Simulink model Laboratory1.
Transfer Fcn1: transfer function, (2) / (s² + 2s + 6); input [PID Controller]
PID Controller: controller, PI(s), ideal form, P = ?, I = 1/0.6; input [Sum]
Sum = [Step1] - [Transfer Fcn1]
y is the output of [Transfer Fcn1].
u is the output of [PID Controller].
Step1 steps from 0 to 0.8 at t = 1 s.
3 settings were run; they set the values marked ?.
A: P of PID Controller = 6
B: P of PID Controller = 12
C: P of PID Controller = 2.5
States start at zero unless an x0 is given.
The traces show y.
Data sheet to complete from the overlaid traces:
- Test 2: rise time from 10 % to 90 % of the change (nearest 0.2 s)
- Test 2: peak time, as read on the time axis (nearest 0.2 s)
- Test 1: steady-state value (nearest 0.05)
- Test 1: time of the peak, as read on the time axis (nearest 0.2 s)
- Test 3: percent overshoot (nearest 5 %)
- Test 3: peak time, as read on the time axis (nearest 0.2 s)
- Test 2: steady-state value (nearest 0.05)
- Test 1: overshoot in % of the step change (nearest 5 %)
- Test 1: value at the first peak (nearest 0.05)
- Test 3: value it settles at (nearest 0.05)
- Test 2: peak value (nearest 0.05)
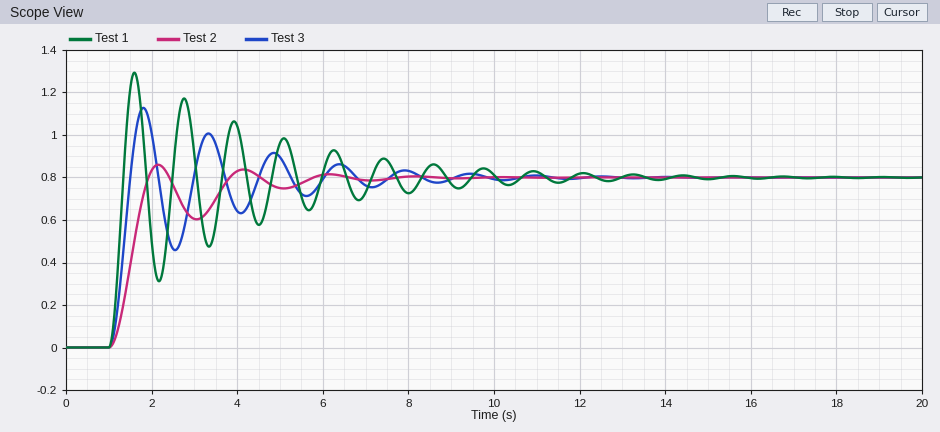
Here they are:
0.6 s
2.2 s
0.80
1.6 s
40 %
1.8 s
0.80
60 %
1.30
0.80
0.85
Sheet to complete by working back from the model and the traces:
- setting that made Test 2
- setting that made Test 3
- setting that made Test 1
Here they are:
C
A
B
